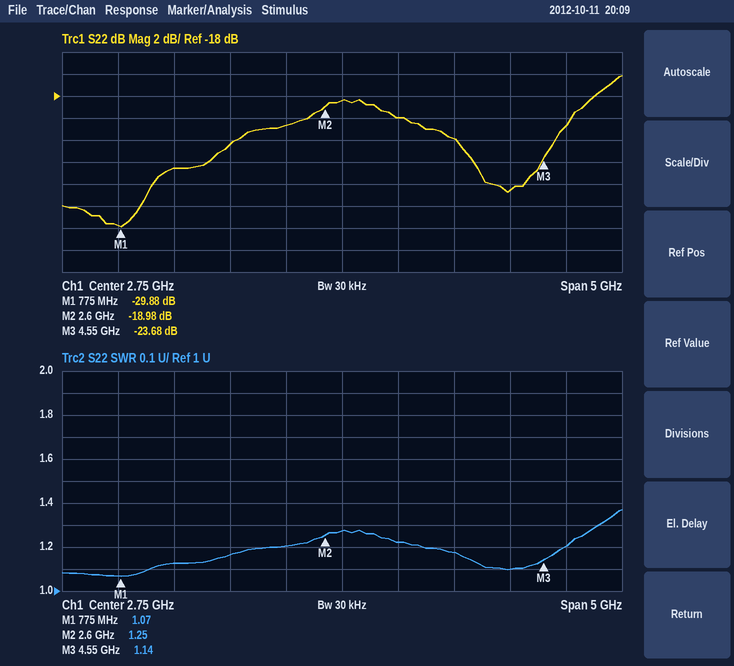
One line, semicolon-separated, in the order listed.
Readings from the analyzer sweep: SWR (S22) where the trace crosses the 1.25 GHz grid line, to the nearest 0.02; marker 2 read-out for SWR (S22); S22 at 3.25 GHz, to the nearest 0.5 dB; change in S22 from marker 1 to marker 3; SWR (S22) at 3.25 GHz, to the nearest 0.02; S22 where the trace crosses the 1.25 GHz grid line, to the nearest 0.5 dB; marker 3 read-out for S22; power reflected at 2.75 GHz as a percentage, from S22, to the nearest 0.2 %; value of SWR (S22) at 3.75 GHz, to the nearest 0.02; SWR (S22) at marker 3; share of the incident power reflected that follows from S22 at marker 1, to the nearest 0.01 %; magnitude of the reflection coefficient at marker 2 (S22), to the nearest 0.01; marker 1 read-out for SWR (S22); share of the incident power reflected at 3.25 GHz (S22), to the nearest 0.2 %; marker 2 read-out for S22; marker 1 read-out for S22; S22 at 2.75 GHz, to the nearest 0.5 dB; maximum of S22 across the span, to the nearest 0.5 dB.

1.12; 1.25; -20.0 dB; 6.20 dB; 1.22; -24.5 dB; -23.68 dB; 1.4 %; 1.18; 1.14; 0.10 %; 0.11; 1.07; 1.0 %; -18.98 dB; -29.88 dB; -18.5 dB; -16.0 dB
